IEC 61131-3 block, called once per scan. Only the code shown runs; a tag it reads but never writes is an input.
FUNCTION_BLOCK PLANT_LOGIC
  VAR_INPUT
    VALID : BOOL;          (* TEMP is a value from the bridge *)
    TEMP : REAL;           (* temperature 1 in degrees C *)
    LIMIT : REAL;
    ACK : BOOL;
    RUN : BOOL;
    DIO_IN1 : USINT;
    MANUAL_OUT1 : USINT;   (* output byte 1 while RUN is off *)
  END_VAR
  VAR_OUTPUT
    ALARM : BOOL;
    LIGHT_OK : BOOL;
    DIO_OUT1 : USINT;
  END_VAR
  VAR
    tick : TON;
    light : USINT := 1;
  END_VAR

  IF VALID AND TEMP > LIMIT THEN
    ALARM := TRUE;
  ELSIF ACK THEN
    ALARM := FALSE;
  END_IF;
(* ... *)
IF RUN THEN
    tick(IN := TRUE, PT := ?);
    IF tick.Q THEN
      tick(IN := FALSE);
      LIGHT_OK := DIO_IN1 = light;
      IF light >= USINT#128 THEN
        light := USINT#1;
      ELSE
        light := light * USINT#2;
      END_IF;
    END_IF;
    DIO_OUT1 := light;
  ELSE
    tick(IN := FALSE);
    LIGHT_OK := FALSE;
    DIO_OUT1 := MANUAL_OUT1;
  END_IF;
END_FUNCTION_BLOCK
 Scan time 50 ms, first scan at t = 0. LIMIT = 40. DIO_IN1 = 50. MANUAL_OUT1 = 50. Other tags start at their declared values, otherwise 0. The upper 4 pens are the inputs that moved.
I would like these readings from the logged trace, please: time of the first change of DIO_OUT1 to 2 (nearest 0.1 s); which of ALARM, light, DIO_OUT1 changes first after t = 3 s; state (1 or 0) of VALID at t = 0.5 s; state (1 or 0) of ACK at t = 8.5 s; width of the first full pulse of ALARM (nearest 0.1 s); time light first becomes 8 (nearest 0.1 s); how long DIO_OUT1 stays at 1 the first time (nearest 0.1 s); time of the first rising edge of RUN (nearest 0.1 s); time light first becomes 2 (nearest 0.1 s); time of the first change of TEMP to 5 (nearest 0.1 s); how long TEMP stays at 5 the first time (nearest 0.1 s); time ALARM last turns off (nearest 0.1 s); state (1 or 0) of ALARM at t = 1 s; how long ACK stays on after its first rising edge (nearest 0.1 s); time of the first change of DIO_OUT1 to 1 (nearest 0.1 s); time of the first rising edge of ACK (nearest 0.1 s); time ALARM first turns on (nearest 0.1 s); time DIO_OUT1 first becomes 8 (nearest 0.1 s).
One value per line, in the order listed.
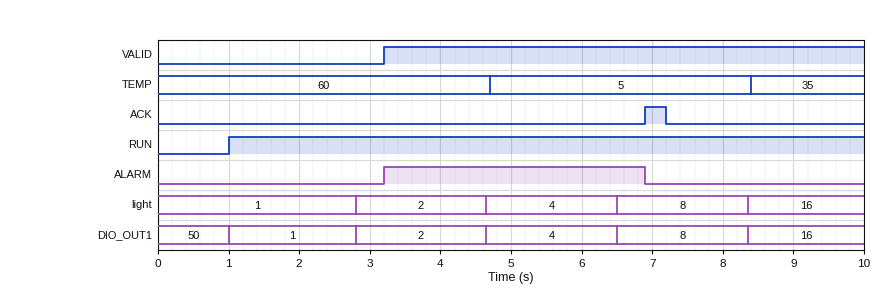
2.8 s
ALARM
0
0
3.7 s
6.5 s
1.8 s
1.0 s
2.8 s
4.7 s
3.7 s
6.9 s
0
0.3 s
1.0 s
6.9 s
3.2 s
6.5 s
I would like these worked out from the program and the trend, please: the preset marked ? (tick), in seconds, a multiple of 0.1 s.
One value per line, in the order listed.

1.8 s
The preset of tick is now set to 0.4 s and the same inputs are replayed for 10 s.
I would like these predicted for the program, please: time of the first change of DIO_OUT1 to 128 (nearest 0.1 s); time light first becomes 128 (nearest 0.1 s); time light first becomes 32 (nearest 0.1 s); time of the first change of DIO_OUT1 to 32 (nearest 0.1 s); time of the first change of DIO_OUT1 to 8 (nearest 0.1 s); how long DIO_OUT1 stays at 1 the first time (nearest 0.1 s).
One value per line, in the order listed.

4.1 s
4.1 s
3.2 s
3.2 s
2.3 s
0.4 s
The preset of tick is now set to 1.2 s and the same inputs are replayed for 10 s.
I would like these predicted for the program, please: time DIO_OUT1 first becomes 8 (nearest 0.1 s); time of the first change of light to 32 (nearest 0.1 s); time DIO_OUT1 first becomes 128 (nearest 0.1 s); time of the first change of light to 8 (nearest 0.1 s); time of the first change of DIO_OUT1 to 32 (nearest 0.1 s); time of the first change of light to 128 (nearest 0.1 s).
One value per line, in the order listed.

4.7 s
7.2 s
9.7 s
4.7 s
7.2 s
9.7 s
